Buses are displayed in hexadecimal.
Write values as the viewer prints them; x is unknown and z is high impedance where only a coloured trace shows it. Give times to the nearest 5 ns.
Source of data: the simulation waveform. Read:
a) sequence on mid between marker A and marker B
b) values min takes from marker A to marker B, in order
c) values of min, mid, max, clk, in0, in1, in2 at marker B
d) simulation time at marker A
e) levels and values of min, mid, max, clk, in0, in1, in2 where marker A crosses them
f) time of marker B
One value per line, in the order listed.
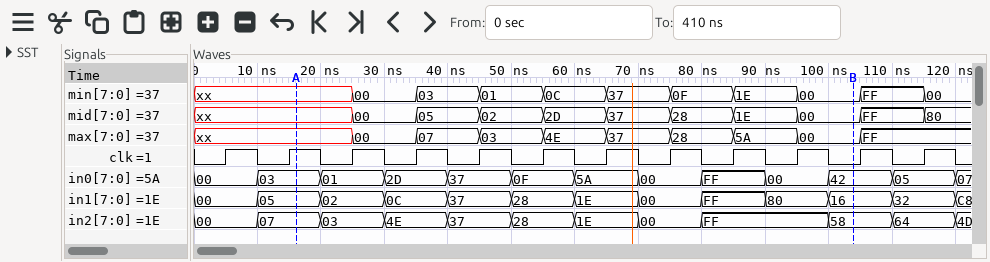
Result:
xx, 00, 05, 02, 2D, 37, 28, 1E, 00
xx, 00, 03, 01, 0C, 37, 0F, 1E, 00
min=00, mid=00, max=00, clk=0, in0=42, in1=16, in2=58
15 ns
min=xx, mid=xx, max=xx, clk=1, in0=03, in1=05, in2=07
105 ns
